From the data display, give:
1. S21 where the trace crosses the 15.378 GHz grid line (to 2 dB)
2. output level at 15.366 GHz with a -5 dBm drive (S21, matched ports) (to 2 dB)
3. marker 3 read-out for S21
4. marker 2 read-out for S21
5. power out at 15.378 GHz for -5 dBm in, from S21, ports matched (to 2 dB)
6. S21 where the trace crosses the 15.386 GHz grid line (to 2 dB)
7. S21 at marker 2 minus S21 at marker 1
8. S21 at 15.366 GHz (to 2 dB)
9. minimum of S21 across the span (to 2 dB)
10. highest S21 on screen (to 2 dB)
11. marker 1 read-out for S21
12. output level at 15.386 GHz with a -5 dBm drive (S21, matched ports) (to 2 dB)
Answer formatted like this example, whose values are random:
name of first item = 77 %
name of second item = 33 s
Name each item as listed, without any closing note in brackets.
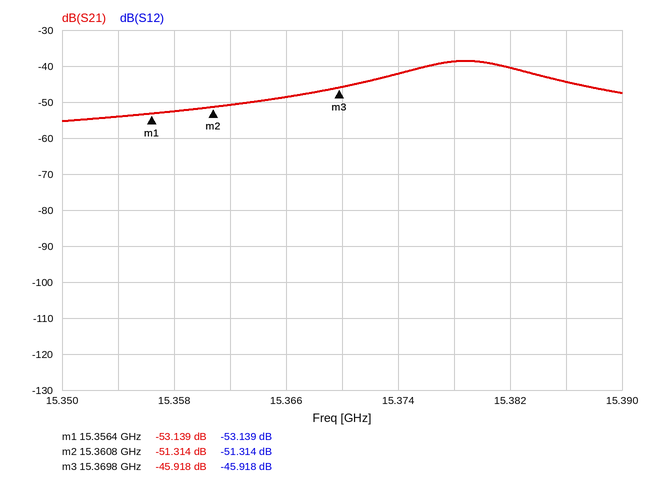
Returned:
S21 where the trace crosses the 15.378 GHz grid line = -38 dB
output level at 15.366 GHz with a -5 dBm drive (S21, matched ports) = -54 dBm
marker 3 read-out for S21 = -45.918 dB
marker 2 read-out for S21 = -51.314 dB
power out at 15.378 GHz for -5 dBm in, from S21, ports matched = -44 dBm
S21 where the trace crosses the 15.386 GHz grid line = -44 dB
S21 at marker 2 minus S21 at marker 1 = 1.825 dB
S21 at 15.366 GHz = -48 dB
minimum of S21 across the span = -56 dB
highest S21 on screen = -38 dB
marker 1 read-out for S21 = -53.139 dB
output level at 15.386 GHz with a -5 dBm drive (S21, matched ports) = -50 dBm
